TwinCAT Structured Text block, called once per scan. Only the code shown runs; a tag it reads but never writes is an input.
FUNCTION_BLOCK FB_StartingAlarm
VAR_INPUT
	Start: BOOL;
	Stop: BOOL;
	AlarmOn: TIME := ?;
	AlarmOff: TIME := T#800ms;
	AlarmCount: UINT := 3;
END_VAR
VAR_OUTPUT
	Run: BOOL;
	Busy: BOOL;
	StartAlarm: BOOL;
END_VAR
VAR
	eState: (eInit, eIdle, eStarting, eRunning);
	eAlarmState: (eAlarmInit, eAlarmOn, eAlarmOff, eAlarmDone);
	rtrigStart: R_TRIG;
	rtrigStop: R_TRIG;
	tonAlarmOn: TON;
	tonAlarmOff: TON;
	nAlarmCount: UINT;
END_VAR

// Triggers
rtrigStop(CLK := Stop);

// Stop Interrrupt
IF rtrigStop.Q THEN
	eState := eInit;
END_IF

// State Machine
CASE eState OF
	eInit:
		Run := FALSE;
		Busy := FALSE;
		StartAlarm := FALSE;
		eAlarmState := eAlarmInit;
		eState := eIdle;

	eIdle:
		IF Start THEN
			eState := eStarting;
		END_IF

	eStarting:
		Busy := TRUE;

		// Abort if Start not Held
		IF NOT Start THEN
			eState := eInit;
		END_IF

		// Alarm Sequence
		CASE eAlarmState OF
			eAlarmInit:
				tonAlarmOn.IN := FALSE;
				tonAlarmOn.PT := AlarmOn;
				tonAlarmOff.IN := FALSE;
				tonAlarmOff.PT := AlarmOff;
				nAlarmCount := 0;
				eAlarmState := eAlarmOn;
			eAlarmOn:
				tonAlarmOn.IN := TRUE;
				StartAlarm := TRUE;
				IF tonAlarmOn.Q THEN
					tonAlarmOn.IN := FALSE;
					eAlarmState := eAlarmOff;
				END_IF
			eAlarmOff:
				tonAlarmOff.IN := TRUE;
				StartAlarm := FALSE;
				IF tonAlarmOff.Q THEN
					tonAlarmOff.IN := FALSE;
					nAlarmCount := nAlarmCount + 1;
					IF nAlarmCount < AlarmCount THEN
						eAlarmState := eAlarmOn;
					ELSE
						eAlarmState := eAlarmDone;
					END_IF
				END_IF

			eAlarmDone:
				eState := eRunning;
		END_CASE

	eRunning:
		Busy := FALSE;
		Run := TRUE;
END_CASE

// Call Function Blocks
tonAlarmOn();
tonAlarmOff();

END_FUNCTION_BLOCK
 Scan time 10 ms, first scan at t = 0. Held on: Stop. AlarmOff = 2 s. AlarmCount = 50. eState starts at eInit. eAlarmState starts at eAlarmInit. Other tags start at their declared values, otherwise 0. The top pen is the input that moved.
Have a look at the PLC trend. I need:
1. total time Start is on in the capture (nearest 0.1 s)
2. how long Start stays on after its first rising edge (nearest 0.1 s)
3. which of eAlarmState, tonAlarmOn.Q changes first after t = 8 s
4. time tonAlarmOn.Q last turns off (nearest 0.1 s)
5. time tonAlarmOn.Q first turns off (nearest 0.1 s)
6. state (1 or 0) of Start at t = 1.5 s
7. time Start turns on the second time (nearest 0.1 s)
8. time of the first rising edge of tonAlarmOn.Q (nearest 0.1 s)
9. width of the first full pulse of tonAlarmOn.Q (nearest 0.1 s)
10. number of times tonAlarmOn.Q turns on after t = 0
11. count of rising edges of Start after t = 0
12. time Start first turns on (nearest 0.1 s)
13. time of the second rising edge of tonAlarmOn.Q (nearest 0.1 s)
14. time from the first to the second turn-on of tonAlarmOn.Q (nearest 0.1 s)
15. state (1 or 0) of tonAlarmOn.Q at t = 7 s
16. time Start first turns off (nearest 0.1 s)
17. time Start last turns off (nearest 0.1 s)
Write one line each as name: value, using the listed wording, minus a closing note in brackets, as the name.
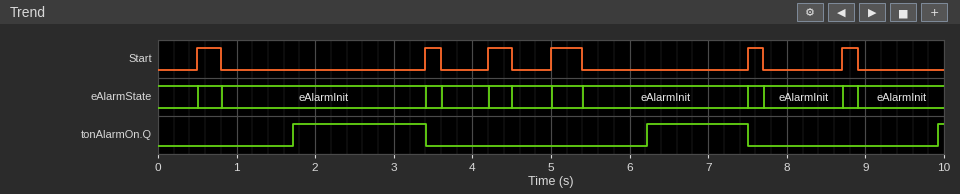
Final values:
total time Start is on in the capture: 1.6 s
how long Start stays on after its first rising edge: 0.3 s
which of eAlarmState, tonAlarmOn.Q changes first after t = 8 s: eAlarmState
time tonAlarmOn.Q last turns off: 7.5 s
time tonAlarmOn.Q first turns off: 3.4 s
state (1 or 0) of Start at t = 1.5 s: 0
time Start turns on the second time: 3.4 s
time of the first rising edge of tonAlarmOn.Q: 1.7 s
width of the first full pulse of tonAlarmOn.Q: 1.7 s
number of times tonAlarmOn.Q turns on after t = 0: 3
count of rising edges of Start after t = 0: 6
time Start first turns on: 0.5 s
time of the second rising edge of tonAlarmOn.Q: 6.2 s
time from the first to the second turn-on of tonAlarmOn.Q: 4.5 s
state (1 or 0) of tonAlarmOn.Q at t = 7 s: 1
time Start first turns off: 0.8 s
time Start last turns off: 8.9 s
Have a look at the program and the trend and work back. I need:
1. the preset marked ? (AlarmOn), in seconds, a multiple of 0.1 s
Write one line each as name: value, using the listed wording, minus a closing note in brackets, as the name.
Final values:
the preset marked ? (AlarmOn), in seconds, a multiple of 0.1 s: 1.2 s
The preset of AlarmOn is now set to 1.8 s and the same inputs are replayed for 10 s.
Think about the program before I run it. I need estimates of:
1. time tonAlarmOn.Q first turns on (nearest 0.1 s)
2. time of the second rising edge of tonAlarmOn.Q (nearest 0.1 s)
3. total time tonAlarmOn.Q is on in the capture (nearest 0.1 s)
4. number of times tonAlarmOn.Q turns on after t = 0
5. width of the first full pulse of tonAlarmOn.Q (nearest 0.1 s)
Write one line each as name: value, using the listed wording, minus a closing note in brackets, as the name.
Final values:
time tonAlarmOn.Q first turns on: 2.3 s
time of the second rising edge of tonAlarmOn.Q: 6.8 s
total time tonAlarmOn.Q is on in the capture: 1.8 s
number of times tonAlarmOn.Q turns on after t = 0: 2
width of the first full pulse of tonAlarmOn.Q: 1.1 s
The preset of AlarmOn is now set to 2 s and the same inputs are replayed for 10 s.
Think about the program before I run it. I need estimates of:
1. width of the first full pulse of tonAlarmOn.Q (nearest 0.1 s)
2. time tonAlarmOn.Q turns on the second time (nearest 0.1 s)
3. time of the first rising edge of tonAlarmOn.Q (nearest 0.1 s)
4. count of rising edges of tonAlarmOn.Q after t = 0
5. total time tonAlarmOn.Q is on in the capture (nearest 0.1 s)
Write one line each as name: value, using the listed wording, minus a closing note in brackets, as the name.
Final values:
width of the first full pulse of tonAlarmOn.Q: 0.9 s
time tonAlarmOn.Q turns on the second time: 7.0 s
time of the first rising edge of tonAlarmOn.Q: 2.5 s
count of rising edges of tonAlarmOn.Q after t = 0: 2
total time tonAlarmOn.Q is on in the capture: 1.4 s
